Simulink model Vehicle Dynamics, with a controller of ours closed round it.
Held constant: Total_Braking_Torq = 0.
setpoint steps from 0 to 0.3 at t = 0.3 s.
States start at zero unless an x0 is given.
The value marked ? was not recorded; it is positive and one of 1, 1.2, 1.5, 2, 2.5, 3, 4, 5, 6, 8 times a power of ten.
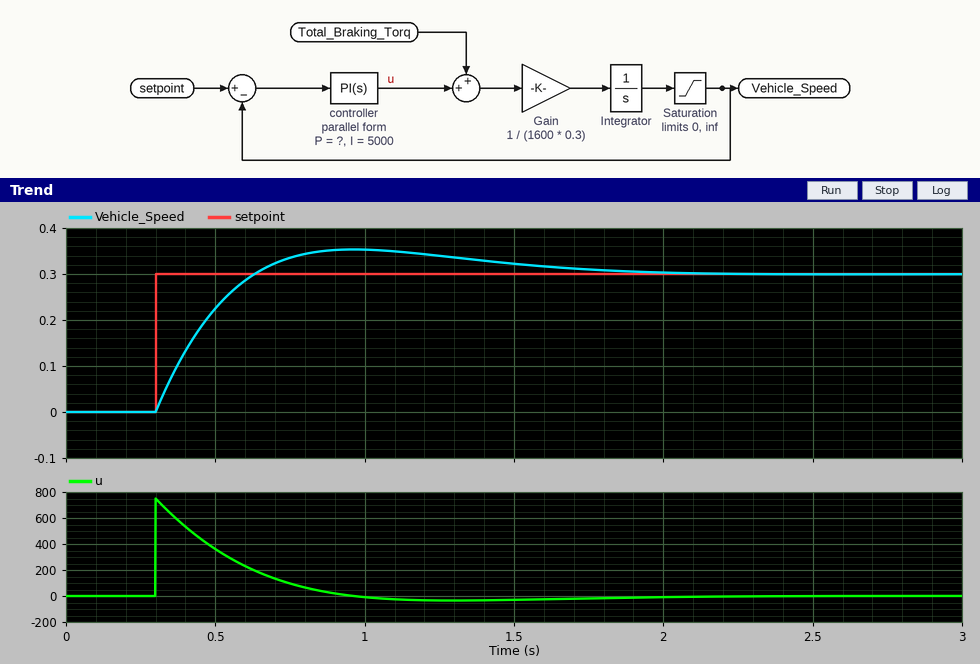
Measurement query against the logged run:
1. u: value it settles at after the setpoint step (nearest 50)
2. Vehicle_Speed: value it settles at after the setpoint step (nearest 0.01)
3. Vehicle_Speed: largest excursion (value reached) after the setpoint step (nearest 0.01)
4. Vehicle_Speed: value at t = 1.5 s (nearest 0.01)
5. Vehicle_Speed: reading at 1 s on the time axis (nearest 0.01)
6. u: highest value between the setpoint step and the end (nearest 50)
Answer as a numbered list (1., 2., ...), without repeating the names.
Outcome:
1. 0
2. 0.30
3. 0.35
4. 0.32
5. 0.35
6. 750
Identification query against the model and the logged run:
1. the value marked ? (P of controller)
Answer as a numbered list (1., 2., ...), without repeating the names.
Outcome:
1. 2500
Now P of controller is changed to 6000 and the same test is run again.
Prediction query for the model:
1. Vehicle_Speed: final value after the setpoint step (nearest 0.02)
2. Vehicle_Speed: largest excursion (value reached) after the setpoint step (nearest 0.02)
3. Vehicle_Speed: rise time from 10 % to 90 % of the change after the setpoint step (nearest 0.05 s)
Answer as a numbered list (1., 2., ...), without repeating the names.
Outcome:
1. 0.30
2. 0.32
3. 0.15 s
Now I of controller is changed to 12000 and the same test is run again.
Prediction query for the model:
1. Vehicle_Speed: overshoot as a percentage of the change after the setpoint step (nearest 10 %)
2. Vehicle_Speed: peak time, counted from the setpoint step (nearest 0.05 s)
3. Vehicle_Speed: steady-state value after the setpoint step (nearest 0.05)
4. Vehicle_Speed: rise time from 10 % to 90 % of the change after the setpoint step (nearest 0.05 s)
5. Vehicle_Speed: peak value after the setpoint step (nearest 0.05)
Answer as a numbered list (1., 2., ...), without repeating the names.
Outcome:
1. 30 %
2. 0.50 s
3. 0.30
4. 0.20 s
5. 0.40
